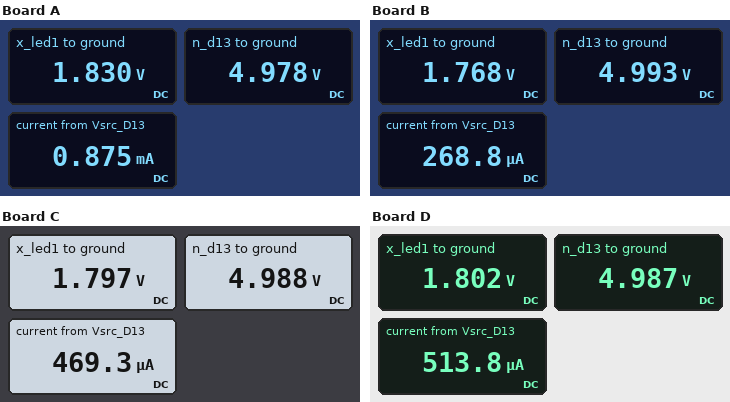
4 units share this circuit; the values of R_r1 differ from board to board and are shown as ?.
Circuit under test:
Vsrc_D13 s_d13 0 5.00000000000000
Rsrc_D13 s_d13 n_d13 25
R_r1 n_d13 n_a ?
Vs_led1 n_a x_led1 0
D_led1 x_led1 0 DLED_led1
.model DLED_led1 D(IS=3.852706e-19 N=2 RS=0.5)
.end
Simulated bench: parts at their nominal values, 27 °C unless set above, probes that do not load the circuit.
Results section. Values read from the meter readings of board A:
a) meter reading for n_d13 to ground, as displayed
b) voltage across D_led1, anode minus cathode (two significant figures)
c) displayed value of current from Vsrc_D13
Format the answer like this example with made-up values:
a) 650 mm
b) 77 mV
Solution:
a) 4.978 V
b) 1.8 V
c) 0.875 mA
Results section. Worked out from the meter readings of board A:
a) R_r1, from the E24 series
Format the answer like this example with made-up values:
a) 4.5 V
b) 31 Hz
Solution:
a) 3.6 kΩ
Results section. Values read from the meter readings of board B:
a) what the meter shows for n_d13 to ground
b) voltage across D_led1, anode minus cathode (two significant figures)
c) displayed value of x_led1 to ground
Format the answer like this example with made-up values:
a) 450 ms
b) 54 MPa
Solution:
a) 4.993 V
b) 1.8 V
c) 1.768 V
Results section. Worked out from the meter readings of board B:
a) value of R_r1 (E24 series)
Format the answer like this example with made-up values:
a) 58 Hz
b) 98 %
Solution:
a) 12 kΩ
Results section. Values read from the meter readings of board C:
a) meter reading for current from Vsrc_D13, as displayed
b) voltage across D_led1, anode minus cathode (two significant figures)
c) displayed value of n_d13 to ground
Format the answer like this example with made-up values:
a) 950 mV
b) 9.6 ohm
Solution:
a) 469.3 µA
b) 1.8 V
c) 4.988 V
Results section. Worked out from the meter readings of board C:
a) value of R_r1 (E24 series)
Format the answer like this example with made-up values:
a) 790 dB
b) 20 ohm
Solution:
a) 6.8 kΩ
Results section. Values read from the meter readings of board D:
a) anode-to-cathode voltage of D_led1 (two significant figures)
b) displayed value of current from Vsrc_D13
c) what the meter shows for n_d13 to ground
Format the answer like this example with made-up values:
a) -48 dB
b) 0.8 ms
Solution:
a) 1.8 V
b) 513.8 µA
c) 4.987 V
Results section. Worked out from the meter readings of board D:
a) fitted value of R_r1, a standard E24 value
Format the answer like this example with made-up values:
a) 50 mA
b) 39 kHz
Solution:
a) 6.2 kΩ
